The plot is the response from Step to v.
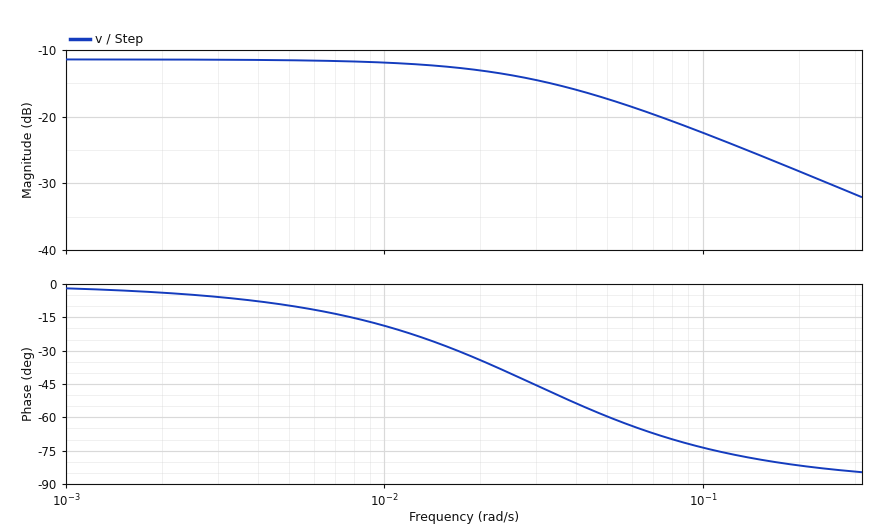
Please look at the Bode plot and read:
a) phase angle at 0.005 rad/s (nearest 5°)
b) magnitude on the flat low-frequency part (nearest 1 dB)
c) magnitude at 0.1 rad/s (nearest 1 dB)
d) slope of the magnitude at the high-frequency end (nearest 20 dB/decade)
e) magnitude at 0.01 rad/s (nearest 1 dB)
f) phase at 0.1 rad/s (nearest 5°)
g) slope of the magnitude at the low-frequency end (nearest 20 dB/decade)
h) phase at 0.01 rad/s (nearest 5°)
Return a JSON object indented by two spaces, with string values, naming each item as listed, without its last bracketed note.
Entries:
{
  "phase angle at 0.005 rad/s": "-10°",
  "magnitude on the flat low-frequency part": "-11 dB",
  "magnitude at 0.1 rad/s": "-22 dB",
  "slope of the magnitude at the high-frequency end": "-20 dB/decade",
  "magnitude at 0.01 rad/s": "-12 dB",
  "phase at 0.1 rad/s": "-75°",
  "slope of the magnitude at the low-frequency end": "0 dB/decade",
  "phase at 0.01 rad/s": "-20°"
}
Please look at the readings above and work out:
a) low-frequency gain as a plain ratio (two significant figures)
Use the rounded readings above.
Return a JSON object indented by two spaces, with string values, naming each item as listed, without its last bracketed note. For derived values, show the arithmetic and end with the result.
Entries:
{
  "low-frequency gain as a plain ratio": "10^(-11 / 20) = 0.28"
}
